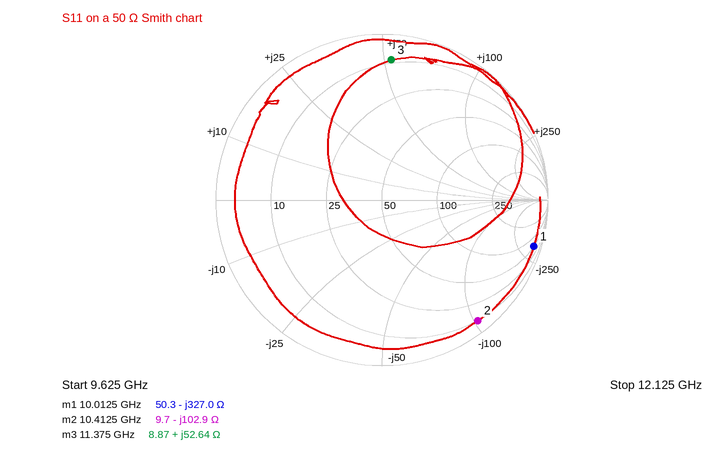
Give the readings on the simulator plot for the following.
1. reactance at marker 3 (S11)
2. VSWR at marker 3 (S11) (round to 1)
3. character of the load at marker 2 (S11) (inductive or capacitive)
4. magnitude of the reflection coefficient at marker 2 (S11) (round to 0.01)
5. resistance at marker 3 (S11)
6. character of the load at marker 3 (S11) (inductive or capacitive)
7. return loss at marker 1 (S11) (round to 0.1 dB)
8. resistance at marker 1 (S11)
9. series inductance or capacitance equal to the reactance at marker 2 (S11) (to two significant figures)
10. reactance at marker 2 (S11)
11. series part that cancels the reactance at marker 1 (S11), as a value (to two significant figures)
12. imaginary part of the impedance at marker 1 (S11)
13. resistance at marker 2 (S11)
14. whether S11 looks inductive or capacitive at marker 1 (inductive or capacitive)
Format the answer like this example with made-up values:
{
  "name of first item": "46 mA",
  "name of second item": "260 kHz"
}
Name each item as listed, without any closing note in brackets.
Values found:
{
  "reactance at marker 3": "+52.64 Ω",
  "VSWR at marker 3 (S11)": "12",
  "character of the load at marker 2 (S11)": "capacitive",
  "magnitude of the reflection coefficient at marker 2 (S11)": "0.93",
  "resistance at marker 3": "8.87 Ω",
  "character of the load at marker 3 (S11)": "inductive",
  "return loss at marker 1 (S11)": "0.4 dB",
  "resistance at marker 1": "50.3 Ω",
  "series inductance or capacitance equal to the reactance at marker 2 (S11)": "150 fF",
  "reactance at marker 2": "-102.9 Ω",
  "series part that cancels the reactance at marker 1 (S11), as a value": "5.2 nH",
  "imaginary part of the impedance at marker 1": "-327.0 Ω",
  "resistance at marker 2": "9.7 Ω",
  "whether S11 looks inductive or capacitive at marker 1": "capacitive"
}
